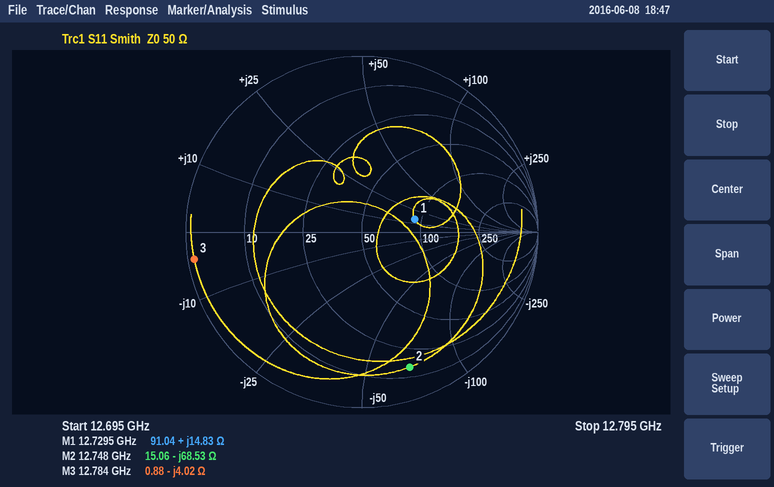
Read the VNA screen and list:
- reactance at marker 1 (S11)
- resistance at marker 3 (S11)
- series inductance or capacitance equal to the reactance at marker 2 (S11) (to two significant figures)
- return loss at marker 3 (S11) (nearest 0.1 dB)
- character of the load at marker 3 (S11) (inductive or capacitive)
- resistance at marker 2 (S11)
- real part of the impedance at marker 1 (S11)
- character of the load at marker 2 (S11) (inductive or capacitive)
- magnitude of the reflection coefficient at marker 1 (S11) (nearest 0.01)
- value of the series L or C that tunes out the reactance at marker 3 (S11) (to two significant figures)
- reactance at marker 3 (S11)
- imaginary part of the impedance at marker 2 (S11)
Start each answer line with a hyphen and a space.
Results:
- +14.83 Ω
- 0.88 Ω
- 180 fF
- 0.3 dB
- capacitive
- 15.06 Ω
- 91.04 Ω
- capacitive
- 0.31
- 50 pH
- -4.02 Ω
- -68.53 Ω
